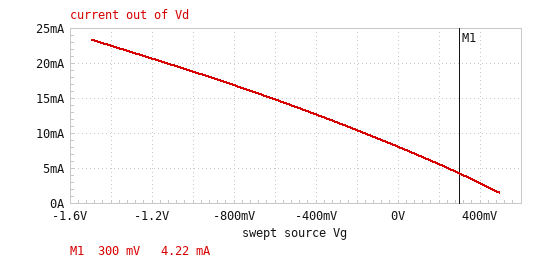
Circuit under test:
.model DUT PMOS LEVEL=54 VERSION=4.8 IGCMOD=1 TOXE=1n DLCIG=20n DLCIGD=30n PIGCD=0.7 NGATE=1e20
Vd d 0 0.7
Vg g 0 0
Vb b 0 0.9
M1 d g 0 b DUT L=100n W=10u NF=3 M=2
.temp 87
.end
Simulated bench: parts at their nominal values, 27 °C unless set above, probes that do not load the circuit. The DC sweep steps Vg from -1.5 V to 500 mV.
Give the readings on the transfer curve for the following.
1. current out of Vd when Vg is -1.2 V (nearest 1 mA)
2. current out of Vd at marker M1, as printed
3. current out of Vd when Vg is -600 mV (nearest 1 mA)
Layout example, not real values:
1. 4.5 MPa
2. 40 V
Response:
1. 21 mA
2. 4.22 mA
3. 15 mA
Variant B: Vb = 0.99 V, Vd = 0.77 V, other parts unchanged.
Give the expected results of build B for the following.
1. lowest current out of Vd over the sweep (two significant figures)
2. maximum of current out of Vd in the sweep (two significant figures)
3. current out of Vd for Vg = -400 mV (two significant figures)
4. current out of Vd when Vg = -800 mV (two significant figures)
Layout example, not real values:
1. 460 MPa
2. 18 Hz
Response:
1. 2.4 mA
2. 25 mA
3. 14 mA
4. 18 mA
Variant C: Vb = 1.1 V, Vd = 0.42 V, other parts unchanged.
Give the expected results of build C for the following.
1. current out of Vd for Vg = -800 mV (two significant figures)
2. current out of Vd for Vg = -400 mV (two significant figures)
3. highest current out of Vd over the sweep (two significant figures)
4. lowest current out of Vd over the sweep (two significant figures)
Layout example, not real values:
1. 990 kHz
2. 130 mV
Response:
1. 11 mA
2. 7.9 mA
3. 15 mA
4. 5.0 µA
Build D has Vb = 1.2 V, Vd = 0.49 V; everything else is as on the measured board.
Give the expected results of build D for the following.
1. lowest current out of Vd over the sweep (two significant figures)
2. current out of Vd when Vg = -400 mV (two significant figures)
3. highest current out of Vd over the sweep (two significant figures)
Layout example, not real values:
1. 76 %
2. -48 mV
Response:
1. 32 µA
2. 9.1 mA
3. 17 mA
